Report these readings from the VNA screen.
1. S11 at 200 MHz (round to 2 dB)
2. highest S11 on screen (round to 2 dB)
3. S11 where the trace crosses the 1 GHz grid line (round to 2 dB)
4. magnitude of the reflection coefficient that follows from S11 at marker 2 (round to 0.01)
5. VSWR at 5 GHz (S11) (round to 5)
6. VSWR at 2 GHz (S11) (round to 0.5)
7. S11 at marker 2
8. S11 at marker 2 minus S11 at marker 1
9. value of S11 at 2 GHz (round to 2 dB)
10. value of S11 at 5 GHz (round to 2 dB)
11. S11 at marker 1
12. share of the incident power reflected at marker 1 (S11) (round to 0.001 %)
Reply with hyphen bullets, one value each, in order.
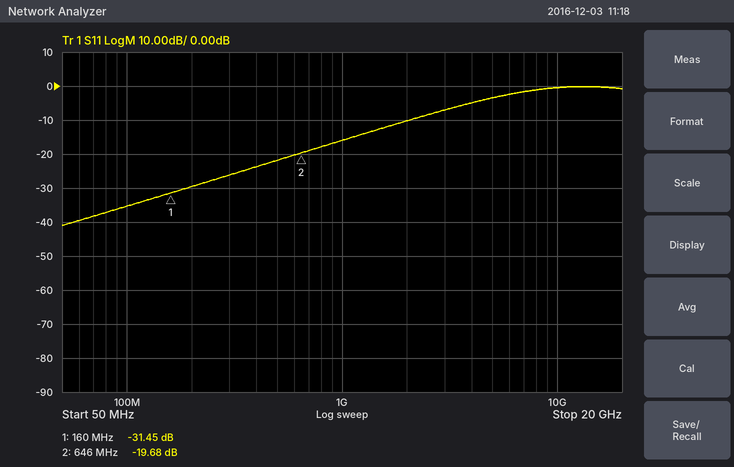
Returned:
- -30 dB
- 0 dB
- -16 dB
- 0.10
- 5
- 2.0
- -19.68 dB
- 11.77 dB
- -10 dB
- -4 dB
- -31.45 dB
- 0.072 %
